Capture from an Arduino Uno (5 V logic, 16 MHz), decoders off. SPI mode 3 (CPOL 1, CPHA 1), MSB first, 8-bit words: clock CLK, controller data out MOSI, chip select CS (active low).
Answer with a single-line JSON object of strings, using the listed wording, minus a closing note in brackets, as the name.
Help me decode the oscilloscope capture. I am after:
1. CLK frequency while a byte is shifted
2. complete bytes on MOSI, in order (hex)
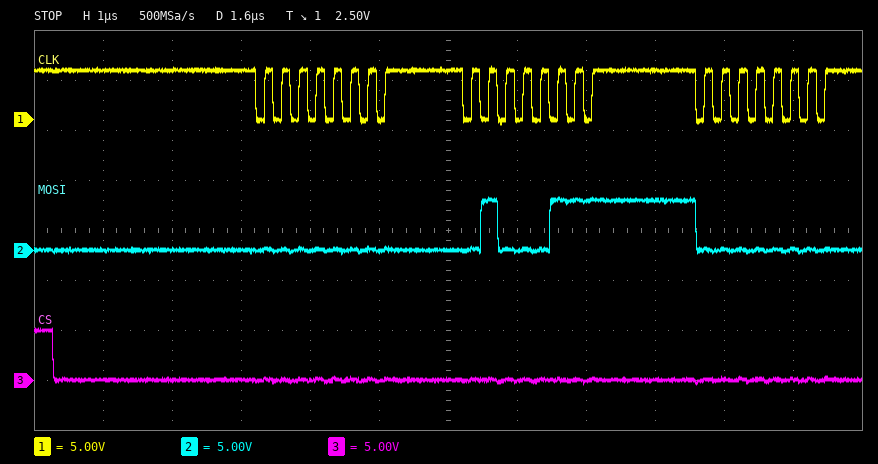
{"CLK frequency while a byte is shifted": "4 MHz", "complete bytes on MOSI, in order": "00 47 00"}
